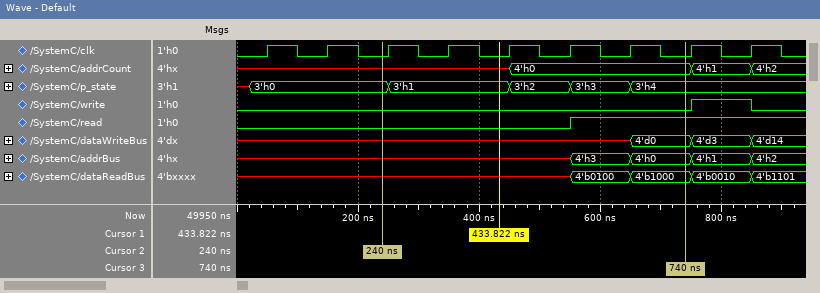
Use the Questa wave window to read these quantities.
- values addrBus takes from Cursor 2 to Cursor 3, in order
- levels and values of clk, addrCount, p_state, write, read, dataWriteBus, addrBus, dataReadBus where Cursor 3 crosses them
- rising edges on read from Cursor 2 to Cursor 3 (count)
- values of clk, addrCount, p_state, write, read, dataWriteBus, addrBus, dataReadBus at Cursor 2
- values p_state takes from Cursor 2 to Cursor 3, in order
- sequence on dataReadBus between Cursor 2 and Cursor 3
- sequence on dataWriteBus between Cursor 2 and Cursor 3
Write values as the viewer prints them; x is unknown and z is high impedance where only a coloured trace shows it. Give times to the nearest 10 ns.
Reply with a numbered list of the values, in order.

1. x, 4'h3, 4'h0
2. clk=0, addrCount=4'h0, p_state=3'h4, write=0, read=1, dataWriteBus=4'd0, addrBus=4'h0, dataReadBus=4'b1000
3. 1
4. clk=0, addrCount=x, p_state=3'h0, write=0, read=0, dataWriteBus=x, addrBus=x, dataReadBus=x
5. 3'h0, 3'h1, 3'h2, 3'h3, 3'h4
6. x, 4'b0100, 4'b1000
7. x, 4'd0
